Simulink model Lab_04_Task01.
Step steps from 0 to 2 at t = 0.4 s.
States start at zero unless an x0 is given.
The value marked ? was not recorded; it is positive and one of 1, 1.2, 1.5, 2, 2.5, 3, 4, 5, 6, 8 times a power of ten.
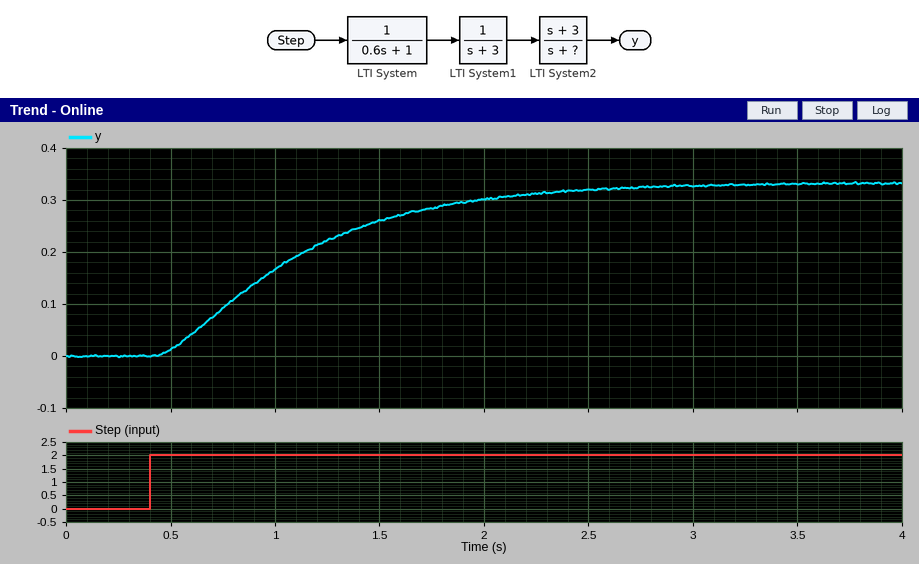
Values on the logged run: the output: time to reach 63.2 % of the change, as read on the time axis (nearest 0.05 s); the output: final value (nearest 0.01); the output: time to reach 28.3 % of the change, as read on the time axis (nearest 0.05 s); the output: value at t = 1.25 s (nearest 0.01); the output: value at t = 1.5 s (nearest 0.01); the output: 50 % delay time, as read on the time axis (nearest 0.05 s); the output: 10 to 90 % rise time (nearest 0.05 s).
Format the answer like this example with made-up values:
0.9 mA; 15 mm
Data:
1.20 s; 0.33; 0.75 s; 0.22; 0.26; 1.00 s; 1.40 s
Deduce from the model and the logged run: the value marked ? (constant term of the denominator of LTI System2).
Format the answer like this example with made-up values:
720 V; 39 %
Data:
6
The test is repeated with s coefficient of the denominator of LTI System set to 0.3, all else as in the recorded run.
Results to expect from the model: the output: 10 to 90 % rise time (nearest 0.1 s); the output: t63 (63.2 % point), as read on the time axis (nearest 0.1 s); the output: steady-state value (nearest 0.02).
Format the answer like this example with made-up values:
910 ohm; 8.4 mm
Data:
0.8 s; 0.9 s; 0.34
